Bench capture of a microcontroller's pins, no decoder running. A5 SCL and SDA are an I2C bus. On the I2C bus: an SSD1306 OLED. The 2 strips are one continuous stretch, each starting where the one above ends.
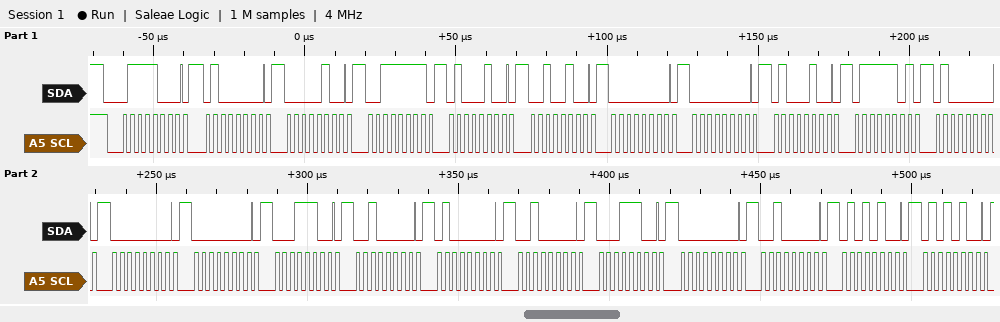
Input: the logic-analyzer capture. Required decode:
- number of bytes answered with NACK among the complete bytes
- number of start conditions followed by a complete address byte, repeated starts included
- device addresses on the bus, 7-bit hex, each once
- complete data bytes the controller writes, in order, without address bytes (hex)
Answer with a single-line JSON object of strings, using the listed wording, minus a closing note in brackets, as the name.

{"number of bytes answered with NACK among the complete bytes": "0", "number of start conditions followed by a complete address byte, repeated starts included": "1", "device addresses on the bus, 7-bit hex, each once": "0x3C", "complete data bytes the controller writes, in order, without address bytes": "40 04 3F 44 24 00 00 44 7D 40 00 00 1C 20 40 20 1C 00 20 54 54"}
